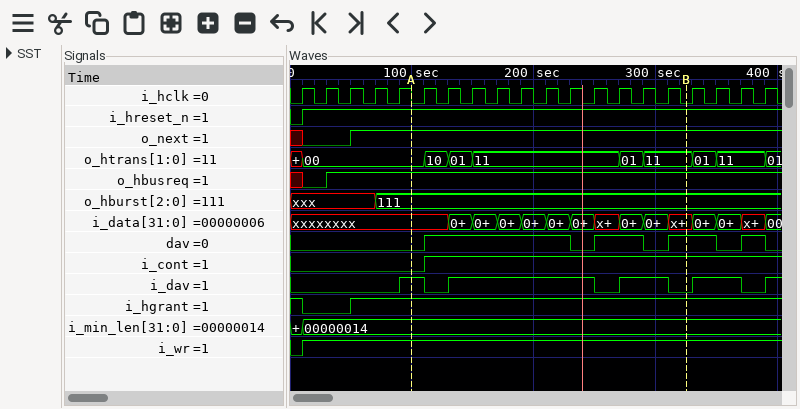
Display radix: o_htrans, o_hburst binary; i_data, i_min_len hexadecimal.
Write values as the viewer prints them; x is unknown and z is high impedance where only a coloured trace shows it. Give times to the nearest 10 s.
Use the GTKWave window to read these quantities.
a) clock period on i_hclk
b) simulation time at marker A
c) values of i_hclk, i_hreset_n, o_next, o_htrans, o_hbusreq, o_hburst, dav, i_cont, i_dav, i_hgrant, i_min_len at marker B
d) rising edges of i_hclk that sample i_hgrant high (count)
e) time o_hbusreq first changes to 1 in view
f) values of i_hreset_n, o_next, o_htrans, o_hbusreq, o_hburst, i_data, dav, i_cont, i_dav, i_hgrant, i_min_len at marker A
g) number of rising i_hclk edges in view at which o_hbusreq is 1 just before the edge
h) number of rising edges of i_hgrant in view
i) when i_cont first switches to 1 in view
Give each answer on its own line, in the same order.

20 s
100 s
i_hclk=0, i_hreset_n=1, o_next=1, o_htrans=11, o_hbusreq=1, o_hburst=111, dav=1, i_cont=1, i_dav=0, i_hgrant=1, i_min_len=00000014
18
30 s
i_hreset_n=1, o_next=1, o_htrans=00, o_hbusreq=1, o_hburst=111, i_data=xxxxxxxx, dav=0, i_cont=0, i_dav=1, i_hgrant=1, i_min_len=00000014
18
1
110 s
